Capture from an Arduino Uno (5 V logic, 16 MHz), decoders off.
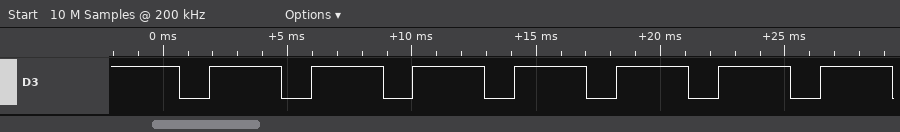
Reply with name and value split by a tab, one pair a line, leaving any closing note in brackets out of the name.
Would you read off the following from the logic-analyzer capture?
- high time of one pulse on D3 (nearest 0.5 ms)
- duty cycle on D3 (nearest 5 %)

high time of one pulse on D3	3.0 ms
duty cycle on D3	70 %
